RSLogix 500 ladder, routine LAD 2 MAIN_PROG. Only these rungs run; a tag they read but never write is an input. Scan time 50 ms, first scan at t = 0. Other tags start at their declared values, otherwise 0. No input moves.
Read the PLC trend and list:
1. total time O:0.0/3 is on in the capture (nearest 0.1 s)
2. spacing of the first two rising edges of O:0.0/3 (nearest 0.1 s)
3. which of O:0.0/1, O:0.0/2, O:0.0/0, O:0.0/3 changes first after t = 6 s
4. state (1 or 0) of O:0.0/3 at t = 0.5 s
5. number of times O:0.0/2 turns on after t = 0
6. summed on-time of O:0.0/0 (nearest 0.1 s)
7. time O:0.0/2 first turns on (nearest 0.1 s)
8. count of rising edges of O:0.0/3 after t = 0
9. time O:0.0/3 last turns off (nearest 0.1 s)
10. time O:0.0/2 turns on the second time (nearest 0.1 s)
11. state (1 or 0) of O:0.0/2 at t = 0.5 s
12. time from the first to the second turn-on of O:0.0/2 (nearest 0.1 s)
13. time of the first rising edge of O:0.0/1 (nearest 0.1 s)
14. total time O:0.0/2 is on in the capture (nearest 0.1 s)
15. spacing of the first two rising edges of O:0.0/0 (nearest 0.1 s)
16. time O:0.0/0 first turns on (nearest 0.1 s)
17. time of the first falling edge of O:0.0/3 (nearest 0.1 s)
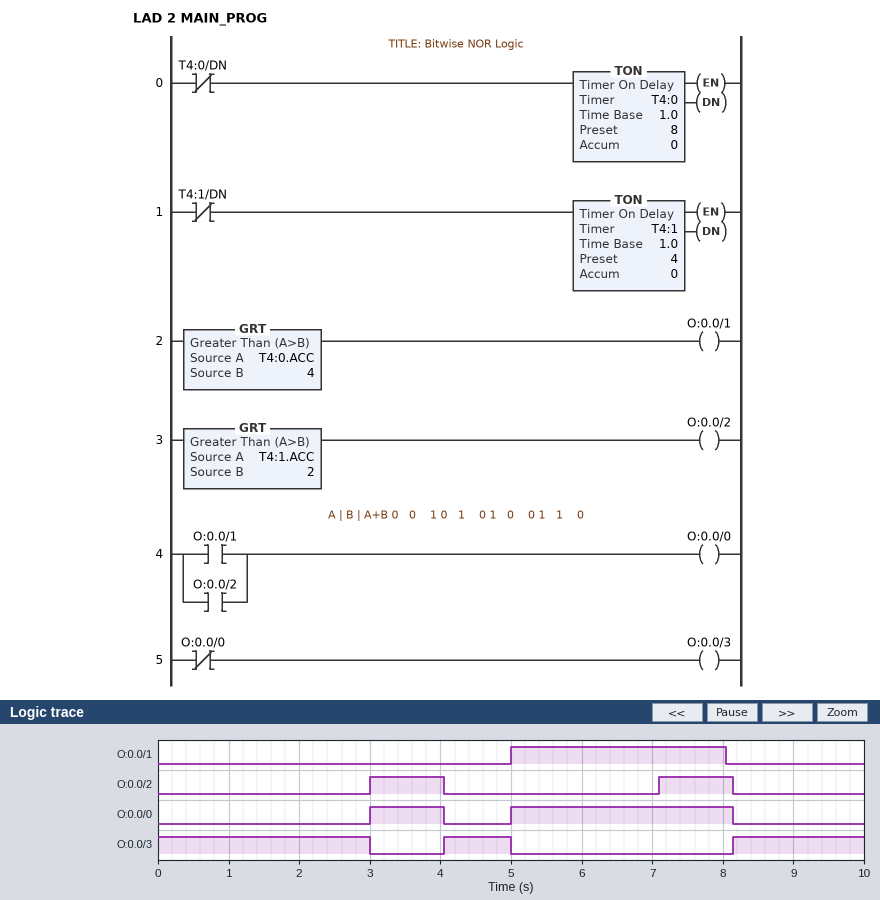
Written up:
5.8 s
4.1 s
O:0.0/2
1
2
4.2 s
3.0 s
2
5.0 s
7.1 s
0
4.1 s
5.0 s
2.1 s
2.0 s
3.0 s
3.0 s
